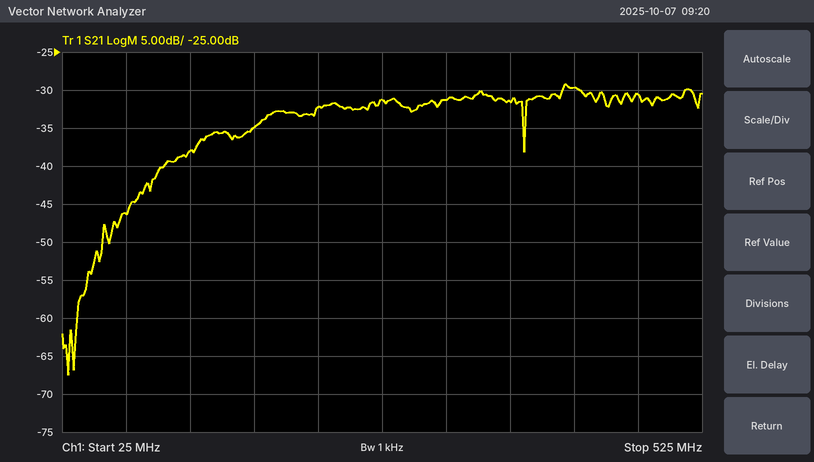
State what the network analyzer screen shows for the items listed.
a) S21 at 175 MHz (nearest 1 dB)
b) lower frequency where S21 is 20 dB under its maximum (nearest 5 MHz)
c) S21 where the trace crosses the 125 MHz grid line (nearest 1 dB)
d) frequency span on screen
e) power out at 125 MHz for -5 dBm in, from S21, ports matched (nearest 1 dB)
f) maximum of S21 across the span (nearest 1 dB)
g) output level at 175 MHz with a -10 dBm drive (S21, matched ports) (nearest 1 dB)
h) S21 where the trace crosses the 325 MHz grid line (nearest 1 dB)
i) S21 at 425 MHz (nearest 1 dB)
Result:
-35 dB
65 MHz
-38 dB
500 MHz
-43 dBm
-29 dB
-45 dBm
-31 dB
-30 dB
